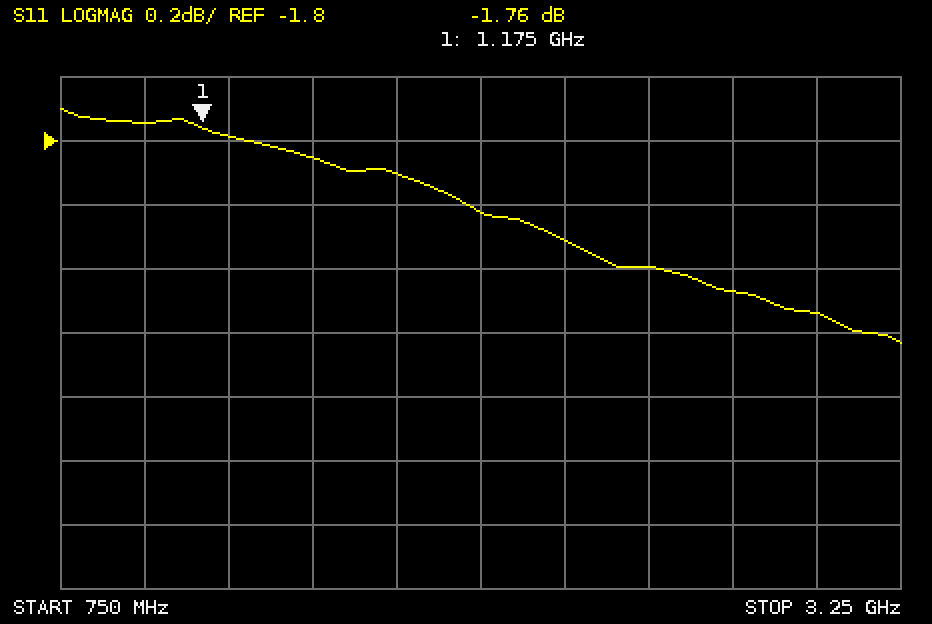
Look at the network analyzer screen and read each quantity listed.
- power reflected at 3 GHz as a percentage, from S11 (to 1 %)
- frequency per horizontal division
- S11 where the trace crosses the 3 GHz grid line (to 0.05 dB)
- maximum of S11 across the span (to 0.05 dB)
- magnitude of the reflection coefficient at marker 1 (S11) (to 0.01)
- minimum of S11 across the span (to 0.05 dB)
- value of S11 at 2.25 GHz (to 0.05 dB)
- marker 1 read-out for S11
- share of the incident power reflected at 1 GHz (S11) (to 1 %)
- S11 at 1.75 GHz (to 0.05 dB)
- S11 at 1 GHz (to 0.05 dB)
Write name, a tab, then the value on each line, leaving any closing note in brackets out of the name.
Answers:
power reflected at 3 GHz as a percentage, from S11	58 %
frequency per horizontal division	250 MHz
S11 where the trace crosses the 3 GHz grid line	-2.35 dB
maximum of S11 across the span	-1.70 dB
magnitude of the reflection coefficient at marker 1 (S11)	0.82
minimum of S11 across the span	-2.45 dB
value of S11 at 2.25 GHz	-2.10 dB
marker 1 read-out for S11	-1.76 dB
share of the incident power reflected at 1 GHz (S11)	67 %
S11 at 1.75 GHz	-1.90 dB
S11 at 1 GHz	-1.75 dB
